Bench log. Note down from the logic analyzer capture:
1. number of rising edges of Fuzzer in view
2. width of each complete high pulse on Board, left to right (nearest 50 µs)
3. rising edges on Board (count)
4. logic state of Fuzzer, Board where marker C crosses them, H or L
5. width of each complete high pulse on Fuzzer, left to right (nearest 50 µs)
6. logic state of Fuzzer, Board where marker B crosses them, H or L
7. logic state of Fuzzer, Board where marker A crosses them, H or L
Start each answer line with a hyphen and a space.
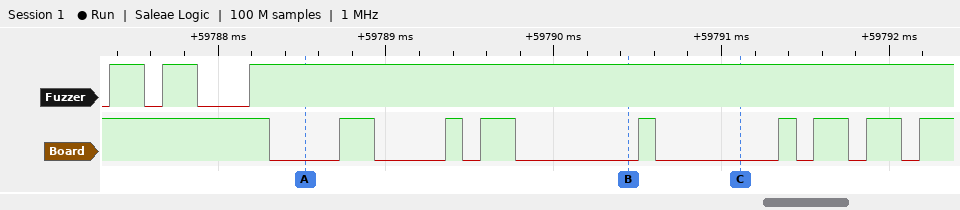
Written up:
- 3
- 200 µs, 100 µs, 200 µs, 100 µs, 100 µs, 200 µs, 200 µs
- 8
- Fuzzer=H, Board=L
- 200 µs, 200 µs
- Fuzzer=H, Board=L
- Fuzzer=H, Board=L
